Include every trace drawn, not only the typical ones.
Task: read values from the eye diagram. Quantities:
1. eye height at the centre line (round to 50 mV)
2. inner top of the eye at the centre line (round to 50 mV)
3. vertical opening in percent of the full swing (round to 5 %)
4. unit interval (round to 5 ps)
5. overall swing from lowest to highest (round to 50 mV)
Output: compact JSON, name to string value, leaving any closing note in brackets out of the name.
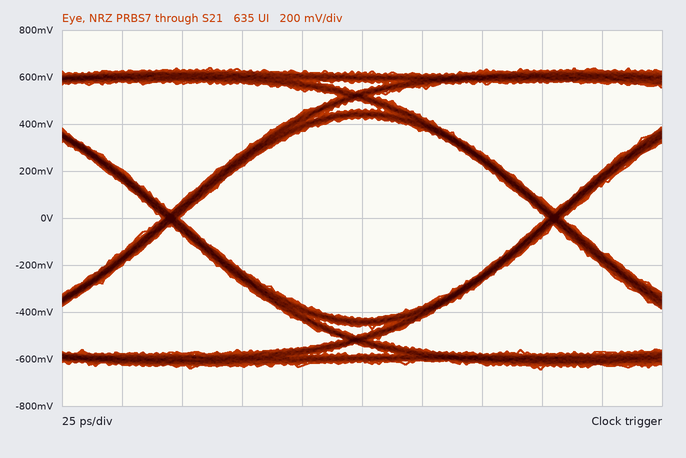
{"eye height at the centre line": "850 mV", "inner top of the eye at the centre line": "450 mV", "vertical opening in percent of the full swing": "65 %", "unit interval": "160 ps", "overall swing from lowest to highest": "1.30 V"}
